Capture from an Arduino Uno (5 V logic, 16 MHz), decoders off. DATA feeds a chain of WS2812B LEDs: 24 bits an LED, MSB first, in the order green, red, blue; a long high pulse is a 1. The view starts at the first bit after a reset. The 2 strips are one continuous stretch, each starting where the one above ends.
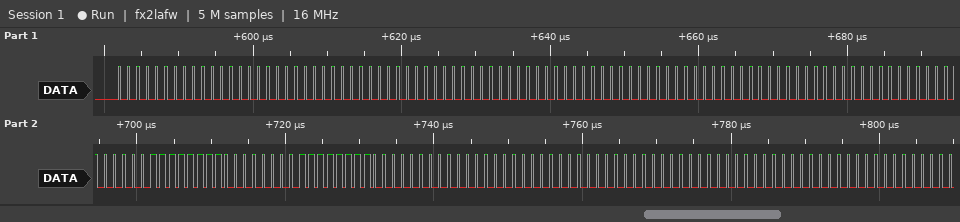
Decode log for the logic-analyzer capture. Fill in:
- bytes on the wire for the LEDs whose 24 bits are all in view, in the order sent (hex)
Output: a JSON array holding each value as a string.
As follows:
["00 00 00 00 00 00 00 00 00 00 00 00 FF 00 FF 00 00 00 00 00 00"]
